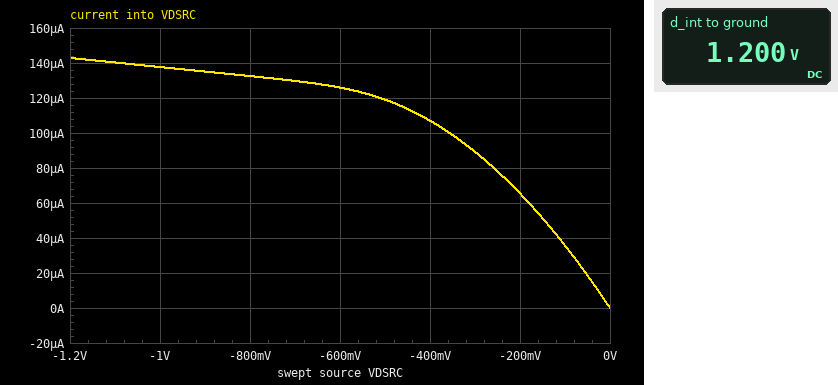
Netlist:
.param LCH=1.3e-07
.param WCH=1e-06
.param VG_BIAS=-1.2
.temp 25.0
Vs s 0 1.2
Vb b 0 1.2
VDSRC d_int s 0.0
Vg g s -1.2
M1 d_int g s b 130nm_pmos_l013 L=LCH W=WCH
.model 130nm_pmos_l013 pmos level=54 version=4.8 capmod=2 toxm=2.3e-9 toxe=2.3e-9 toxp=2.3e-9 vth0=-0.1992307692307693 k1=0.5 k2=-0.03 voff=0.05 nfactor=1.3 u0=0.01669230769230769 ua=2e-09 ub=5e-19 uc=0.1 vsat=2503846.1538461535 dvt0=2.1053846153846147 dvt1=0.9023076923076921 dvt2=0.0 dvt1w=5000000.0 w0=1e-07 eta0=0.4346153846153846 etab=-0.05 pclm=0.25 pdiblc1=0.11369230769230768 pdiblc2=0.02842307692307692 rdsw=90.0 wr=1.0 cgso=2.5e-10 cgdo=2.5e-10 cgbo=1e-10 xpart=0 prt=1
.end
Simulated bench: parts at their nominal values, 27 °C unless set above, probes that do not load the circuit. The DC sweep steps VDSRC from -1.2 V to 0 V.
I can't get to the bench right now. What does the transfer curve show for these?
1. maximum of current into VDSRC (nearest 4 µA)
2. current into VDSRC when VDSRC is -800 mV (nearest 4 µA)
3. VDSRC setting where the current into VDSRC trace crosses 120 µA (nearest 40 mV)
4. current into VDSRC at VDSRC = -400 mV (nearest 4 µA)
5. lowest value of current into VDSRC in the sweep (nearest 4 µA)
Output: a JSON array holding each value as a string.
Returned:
["144 µA", "132 µA", "-520 mV", "108 µA", "0 A"]
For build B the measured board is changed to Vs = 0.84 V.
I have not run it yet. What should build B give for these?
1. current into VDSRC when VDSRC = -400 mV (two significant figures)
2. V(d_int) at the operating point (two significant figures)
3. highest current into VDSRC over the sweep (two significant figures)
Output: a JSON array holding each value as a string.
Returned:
["1.7 mA", "840 mV", "2.4 mA"]
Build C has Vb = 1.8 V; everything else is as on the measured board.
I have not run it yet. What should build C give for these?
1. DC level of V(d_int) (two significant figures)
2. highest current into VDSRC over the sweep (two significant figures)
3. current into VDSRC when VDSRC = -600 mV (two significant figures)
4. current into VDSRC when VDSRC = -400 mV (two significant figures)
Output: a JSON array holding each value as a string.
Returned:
["1.2 V", "2.2 mA", "1.8 mA", "1.6 mA"]
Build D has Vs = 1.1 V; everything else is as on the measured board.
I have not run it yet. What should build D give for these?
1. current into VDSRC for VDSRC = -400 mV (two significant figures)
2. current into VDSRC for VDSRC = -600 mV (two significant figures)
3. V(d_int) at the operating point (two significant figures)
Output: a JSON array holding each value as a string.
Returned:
["1.9 mA", "2.3 mA", "1.1 V"]
